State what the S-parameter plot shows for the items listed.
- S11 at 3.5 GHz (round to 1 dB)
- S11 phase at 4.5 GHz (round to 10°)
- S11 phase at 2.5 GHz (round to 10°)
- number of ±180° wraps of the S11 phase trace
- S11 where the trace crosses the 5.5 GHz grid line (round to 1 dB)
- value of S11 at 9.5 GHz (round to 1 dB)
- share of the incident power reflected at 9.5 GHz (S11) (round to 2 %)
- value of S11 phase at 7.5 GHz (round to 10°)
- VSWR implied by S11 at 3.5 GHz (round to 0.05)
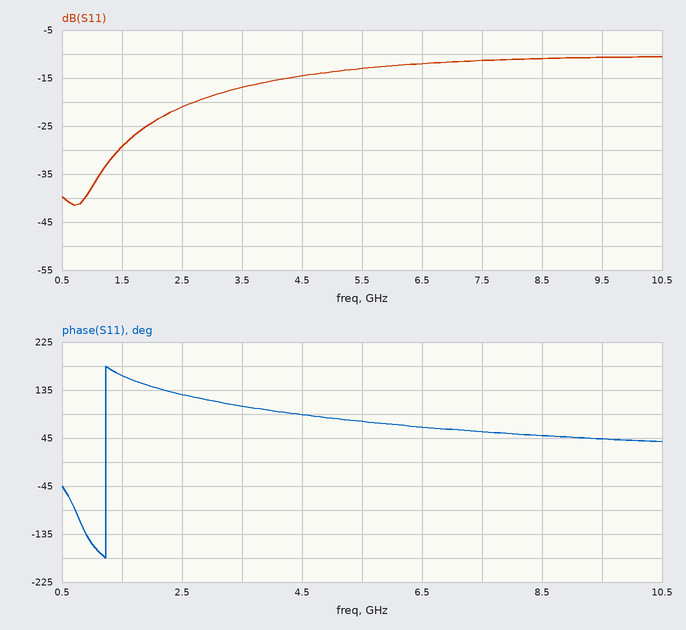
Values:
-17 dB
90°
130°
1
-13 dB
-11 dB
8 %
60°
1.35
